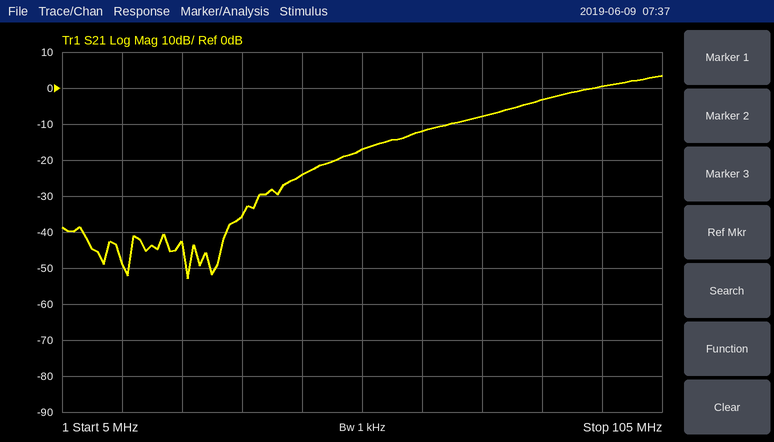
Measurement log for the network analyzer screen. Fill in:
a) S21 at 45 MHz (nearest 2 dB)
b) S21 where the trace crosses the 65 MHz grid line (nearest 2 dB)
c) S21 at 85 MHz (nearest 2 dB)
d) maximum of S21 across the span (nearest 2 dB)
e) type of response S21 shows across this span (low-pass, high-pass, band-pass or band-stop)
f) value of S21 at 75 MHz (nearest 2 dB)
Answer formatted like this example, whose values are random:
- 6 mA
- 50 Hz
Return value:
- -24 dB
- -12 dB
- -4 dB
- 4 dB
- high-pass
- -8 dB
